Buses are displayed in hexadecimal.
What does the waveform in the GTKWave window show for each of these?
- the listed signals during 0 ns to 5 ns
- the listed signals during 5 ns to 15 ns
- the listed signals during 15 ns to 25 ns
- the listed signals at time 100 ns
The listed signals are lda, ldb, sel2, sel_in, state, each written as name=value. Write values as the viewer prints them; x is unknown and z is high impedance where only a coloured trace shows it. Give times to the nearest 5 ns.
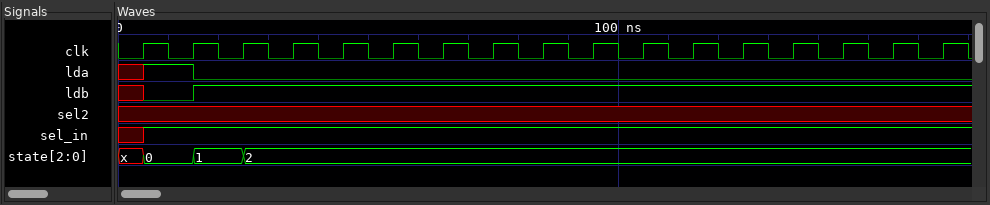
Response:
lda=x, ldb=x, sel2=x, sel_in=x, state=x
lda=1, ldb=0, sel2=x, sel_in=1, state=0
lda=0, ldb=1, sel2=x, sel_in=1, state=1
lda=0, ldb=1, sel2=x, sel_in=1, state=2
